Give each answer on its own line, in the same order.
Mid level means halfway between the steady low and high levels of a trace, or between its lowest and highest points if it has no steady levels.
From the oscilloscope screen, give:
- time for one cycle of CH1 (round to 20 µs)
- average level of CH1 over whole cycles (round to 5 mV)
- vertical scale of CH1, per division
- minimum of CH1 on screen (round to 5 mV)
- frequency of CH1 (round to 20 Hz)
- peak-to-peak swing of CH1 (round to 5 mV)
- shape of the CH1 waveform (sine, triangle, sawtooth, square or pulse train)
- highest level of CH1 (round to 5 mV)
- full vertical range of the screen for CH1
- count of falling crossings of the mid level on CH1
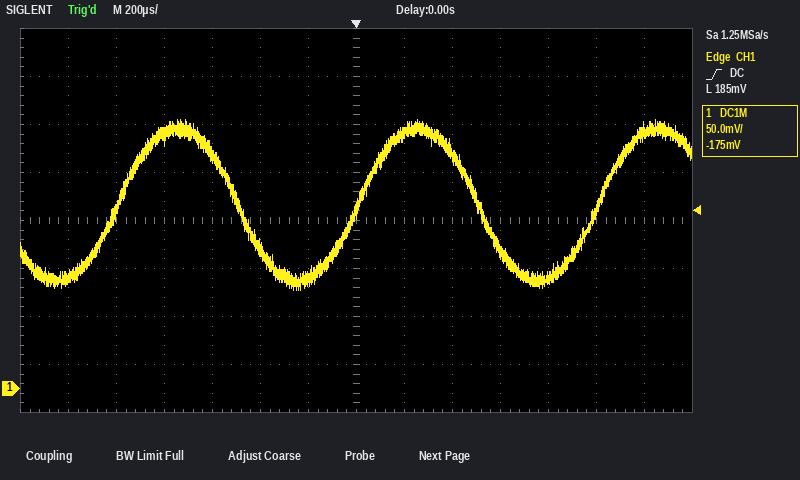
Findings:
1.00 ms
190 mV
50 mV
100 mV
1.00 kHz
180 mV
sine
280 mV
400 mV
2
